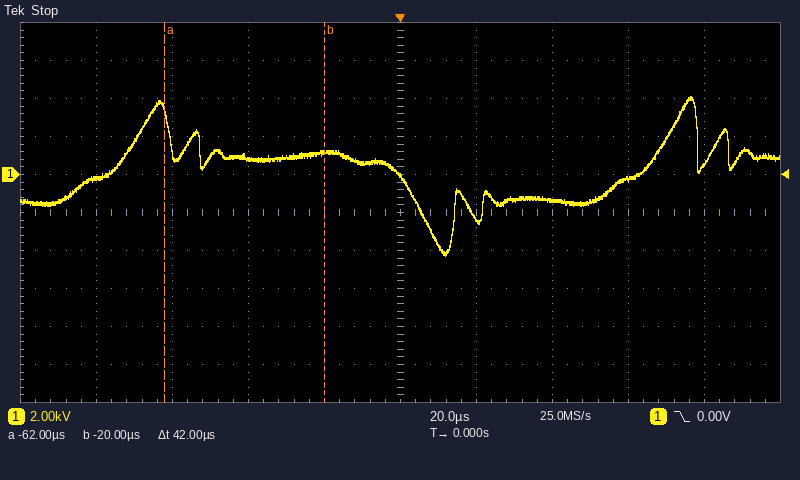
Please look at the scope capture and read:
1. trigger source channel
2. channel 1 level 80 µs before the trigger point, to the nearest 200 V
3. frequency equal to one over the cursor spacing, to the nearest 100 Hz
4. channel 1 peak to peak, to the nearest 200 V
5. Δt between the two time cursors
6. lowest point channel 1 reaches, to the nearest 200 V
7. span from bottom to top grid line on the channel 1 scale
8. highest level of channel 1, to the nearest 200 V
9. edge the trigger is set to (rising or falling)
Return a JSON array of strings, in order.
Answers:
["channel 1", "-200 V", "23.8 kHz", "8.4 kV", "42 µs", "-4.2 kV", "20 kV", "4.2 kV", "falling"]
